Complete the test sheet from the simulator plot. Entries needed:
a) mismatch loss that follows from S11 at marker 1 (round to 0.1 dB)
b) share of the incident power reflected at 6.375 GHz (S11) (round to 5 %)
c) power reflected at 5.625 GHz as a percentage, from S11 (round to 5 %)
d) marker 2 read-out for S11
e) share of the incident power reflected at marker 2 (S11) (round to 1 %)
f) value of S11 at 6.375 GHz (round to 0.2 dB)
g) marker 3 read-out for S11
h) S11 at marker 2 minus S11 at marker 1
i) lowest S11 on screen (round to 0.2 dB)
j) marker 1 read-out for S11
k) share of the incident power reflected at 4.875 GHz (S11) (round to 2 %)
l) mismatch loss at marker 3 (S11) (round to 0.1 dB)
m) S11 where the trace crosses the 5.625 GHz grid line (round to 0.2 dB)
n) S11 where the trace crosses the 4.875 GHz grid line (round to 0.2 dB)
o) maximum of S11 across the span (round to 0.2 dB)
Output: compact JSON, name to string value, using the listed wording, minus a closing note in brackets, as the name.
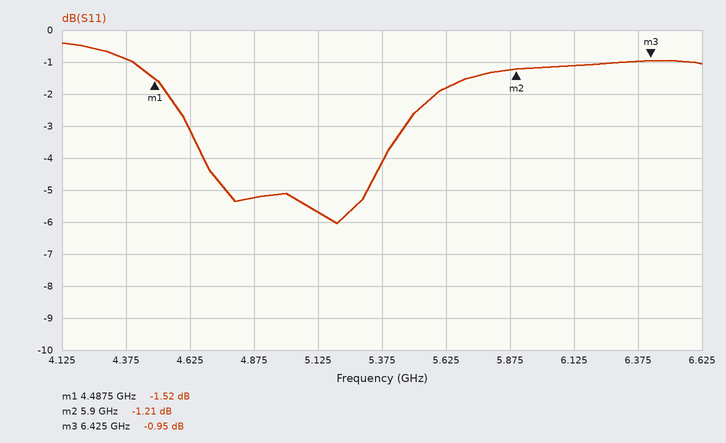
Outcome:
{"mismatch loss that follows from S11 at marker 1": "5.3 dB", "share of the incident power reflected at 6.375 GHz (S11)": "80 %", "power reflected at 5.625 GHz as a percentage, from S11": "65 %", "marker 2 read-out for S11": "-1.21 dB", "share of the incident power reflected at marker 2 (S11)": "76 %", "value of S11 at 6.375 GHz": "-1.0 dB", "marker 3 read-out for S11": "-0.95 dB", "S11 at marker 2 minus S11 at marker 1": "0.31 dB", "lowest S11 on screen": "-6.0 dB", "marker 1 read-out for S11": "-1.52 dB", "share of the incident power reflected at 4.875 GHz (S11)": "30 %", "mismatch loss at marker 3 (S11)": "7.1 dB", "S11 where the trace crosses the 5.625 GHz grid line": "-1.8 dB", "S11 where the trace crosses the 4.875 GHz grid line": "-5.2 dB", "maximum of S11 across the span": "-0.4 dB"}
